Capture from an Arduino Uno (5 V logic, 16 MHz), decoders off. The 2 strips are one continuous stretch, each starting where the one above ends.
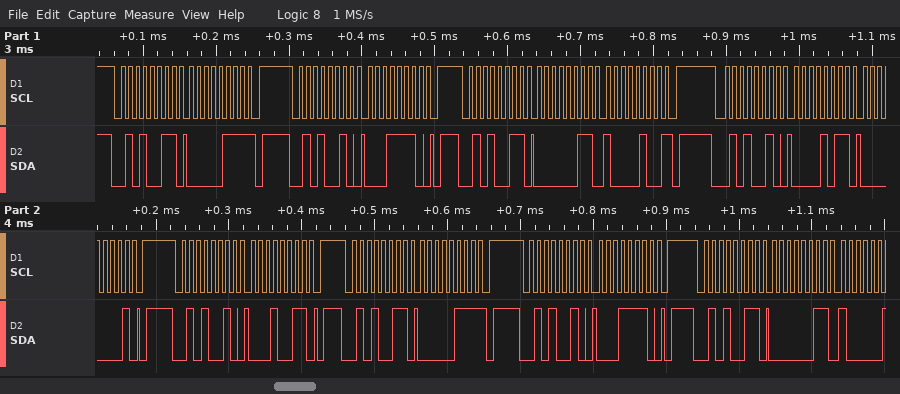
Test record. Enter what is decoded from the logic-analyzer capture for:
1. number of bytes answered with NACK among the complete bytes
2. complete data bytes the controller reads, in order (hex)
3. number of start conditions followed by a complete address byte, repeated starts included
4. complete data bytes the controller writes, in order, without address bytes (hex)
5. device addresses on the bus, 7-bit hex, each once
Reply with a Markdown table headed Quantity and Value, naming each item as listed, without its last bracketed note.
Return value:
| Quantity | Value |
|---|---|
| number of bytes answered with NACK among the complete bytes | 3 |
| complete data bytes the controller reads, in order | 07 03 84 07 03 |
| number of start conditions followed by a complete address byte, repeated starts included | 8 |
| complete data bytes the controller writes, in order, without address bytes | 1E 0B 01 13 1E |
| device addresses on the bus, 7-bit hex, each once | 0x29 |
